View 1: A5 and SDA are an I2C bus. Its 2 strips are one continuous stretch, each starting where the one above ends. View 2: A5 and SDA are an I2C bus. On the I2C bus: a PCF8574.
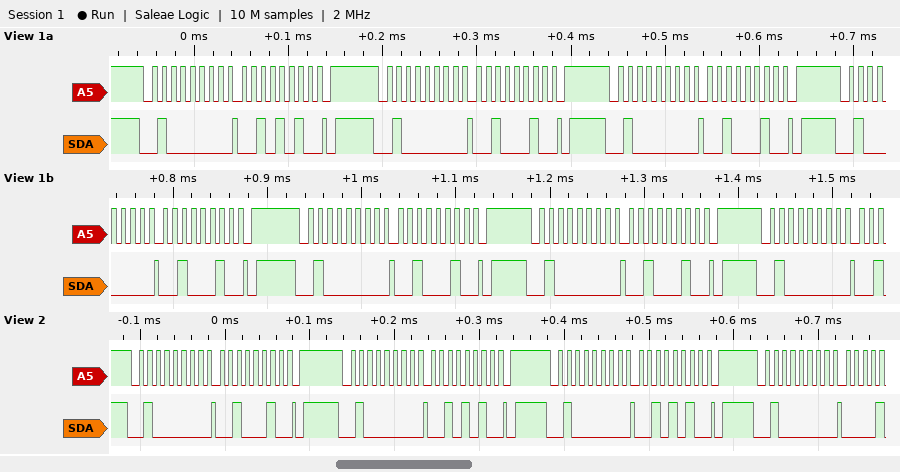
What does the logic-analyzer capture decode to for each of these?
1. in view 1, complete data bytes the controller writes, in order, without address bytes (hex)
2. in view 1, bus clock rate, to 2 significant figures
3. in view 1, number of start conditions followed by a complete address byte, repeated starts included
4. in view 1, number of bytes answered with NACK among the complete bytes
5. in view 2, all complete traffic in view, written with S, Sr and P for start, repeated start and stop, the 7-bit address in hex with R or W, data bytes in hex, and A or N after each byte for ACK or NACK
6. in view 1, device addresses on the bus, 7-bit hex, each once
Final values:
2A 22 22 22 22 22
100 kHz
7
0
S 20W A 22 A P S 20W A 2A A P S 20W A 2A A P S 20W A
0x20
